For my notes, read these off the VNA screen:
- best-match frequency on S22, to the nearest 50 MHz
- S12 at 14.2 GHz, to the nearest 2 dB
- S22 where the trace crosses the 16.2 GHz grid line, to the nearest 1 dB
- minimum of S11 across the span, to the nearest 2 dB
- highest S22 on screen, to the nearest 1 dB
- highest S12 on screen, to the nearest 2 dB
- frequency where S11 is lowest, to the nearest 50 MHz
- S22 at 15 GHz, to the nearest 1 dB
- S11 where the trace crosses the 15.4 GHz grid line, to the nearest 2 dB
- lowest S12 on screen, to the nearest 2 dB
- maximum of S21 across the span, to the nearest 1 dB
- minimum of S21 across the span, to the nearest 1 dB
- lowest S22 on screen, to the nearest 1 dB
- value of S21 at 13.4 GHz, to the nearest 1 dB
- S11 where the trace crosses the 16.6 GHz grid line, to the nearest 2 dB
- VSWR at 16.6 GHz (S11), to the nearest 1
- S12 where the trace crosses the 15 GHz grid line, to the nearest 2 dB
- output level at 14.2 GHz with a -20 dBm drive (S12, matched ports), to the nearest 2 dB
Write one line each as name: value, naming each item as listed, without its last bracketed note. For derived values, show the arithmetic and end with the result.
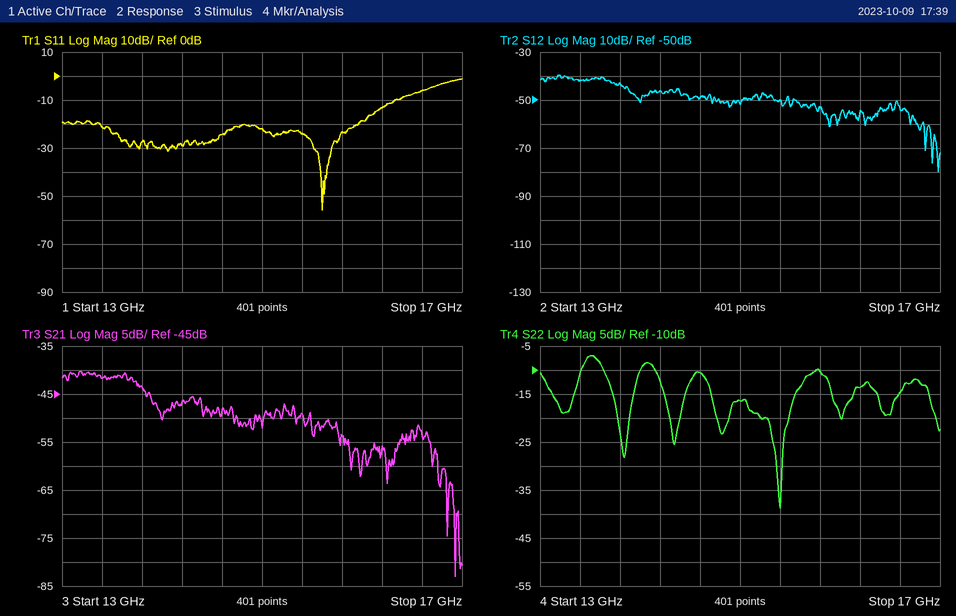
best-match frequency on S22, to the nearest 50 MHz: 15.40 GHz
S12 at 14.2 GHz, to the nearest 2 dB: -46 dB
S22 where the trace crosses the 16.2 GHz grid line, to the nearest 1 dB: -14 dB
minimum of S11 across the span, to the nearest 2 dB: -56 dB
highest S22 on screen, to the nearest 1 dB: -7 dB
highest S12 on screen, to the nearest 2 dB: -40 dB
frequency where S11 is lowest, to the nearest 50 MHz: 15.60 GHz
S22 at 15 GHz, to the nearest 1 dB: -16 dB
S11 where the trace crosses the 15.4 GHz grid line, to the nearest 2 dB: -24 dB
lowest S12 on screen, to the nearest 2 dB: -80 dB
maximum of S21 across the span, to the nearest 1 dB: -40 dB
minimum of S21 across the span, to the nearest 1 dB: -83 dB
lowest S22 on screen, to the nearest 1 dB: -39 dB
value of S21 at 13.4 GHz, to the nearest 1 dB: -42 dB
S11 where the trace crosses the 16.6 GHz grid line, to the nearest 2 dB: -6 dB
VSWR at 16.6 GHz (S11), to the nearest 1: |Γ| = 10^(-6/20) = 0.5012; VSWR = (1 + 0.5012)/(1 − 0.5012) ≈ 3
S12 where the trace crosses the 15 GHz grid line, to the nearest 2 dB: -52 dB
output level at 14.2 GHz with a -20 dBm drive (S12, matched ports), to the nearest 2 dB: -20 dBm + (-46 dB) = -66 dBm
